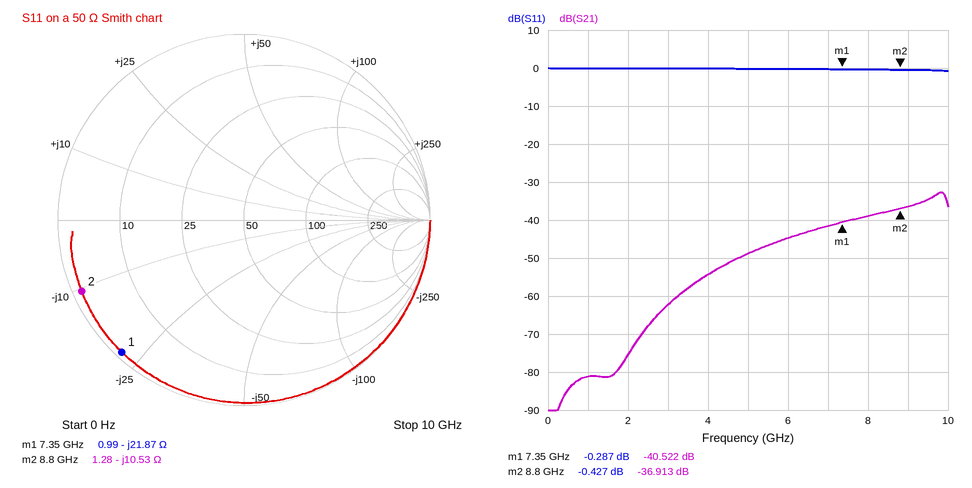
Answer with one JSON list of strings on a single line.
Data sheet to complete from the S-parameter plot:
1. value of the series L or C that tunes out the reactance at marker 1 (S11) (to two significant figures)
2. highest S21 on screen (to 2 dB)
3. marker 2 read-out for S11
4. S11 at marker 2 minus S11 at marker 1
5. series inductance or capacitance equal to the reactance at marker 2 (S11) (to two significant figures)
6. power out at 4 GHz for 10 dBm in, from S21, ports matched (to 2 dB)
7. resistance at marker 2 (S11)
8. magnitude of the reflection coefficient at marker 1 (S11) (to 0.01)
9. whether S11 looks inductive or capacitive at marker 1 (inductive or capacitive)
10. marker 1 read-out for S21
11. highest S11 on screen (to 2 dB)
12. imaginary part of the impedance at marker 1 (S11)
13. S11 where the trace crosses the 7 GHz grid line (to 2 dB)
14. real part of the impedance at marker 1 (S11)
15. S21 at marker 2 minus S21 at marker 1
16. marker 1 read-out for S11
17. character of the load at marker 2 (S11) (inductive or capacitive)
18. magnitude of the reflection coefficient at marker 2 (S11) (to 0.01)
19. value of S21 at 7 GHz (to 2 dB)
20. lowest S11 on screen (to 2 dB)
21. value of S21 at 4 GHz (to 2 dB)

["470 pH", "-32 dB", "-0.427 dB", "-0.140 dB", "1.7 pF", "-44 dBm", "1.28 Ω", "0.97", "capacitive", "-40.522 dB", "0 dB", "-21.87 Ω", "0 dB", "0.99 Ω", "3.609 dB", "-0.287 dB", "capacitive", "0.95", "-42 dB", "0 dB", "-54 dB"]
